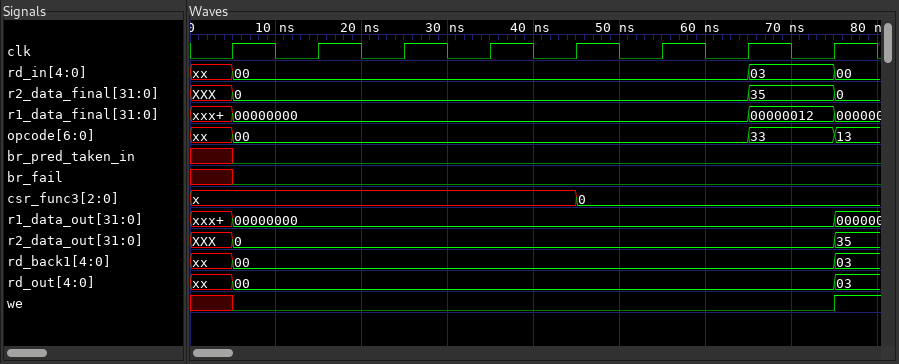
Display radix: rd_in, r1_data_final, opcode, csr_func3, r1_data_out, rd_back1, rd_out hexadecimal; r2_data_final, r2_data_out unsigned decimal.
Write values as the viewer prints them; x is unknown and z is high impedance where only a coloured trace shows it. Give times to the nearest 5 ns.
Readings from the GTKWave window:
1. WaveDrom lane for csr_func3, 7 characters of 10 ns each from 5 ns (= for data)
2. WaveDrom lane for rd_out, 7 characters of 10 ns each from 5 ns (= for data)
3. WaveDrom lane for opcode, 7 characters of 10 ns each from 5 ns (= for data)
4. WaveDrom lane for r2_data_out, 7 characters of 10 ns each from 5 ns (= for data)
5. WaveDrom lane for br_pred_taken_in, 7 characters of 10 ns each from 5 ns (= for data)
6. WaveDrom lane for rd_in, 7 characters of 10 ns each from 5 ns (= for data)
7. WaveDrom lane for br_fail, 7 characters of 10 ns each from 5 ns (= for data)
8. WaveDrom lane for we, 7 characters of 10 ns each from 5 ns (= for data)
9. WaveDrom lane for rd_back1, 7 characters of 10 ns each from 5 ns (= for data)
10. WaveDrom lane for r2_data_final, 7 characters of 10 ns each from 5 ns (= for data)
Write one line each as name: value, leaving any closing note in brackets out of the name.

WaveDrom lane for csr_func3, 7 characters of 10 ns each from 5 ns: {name: 'csr_func3', wave: 'x...=..', data: '0'}
WaveDrom lane for rd_out, 7 characters of 10 ns each from 5 ns: {name: 'rd_out', wave: '=......', data: '00'}
WaveDrom lane for opcode, 7 characters of 10 ns each from 5 ns: {name: 'opcode', wave: '=.....=', data: '00 33'}
WaveDrom lane for r2_data_out, 7 characters of 10 ns each from 5 ns: {name: 'r2_data_out', wave: '=......', data: '0'}
WaveDrom lane for br_pred_taken_in, 7 characters of 10 ns each from 5 ns: {name: 'br_pred_taken_in', wave: '0......'}
WaveDrom lane for rd_in, 7 characters of 10 ns each from 5 ns: {name: 'rd_in', wave: '=.....=', data: '00 03'}
WaveDrom lane for br_fail, 7 characters of 10 ns each from 5 ns: {name: 'br_fail', wave: '0......'}
WaveDrom lane for we, 7 characters of 10 ns each from 5 ns: {name: 'we', wave: '0......'}
WaveDrom lane for rd_back1, 7 characters of 10 ns each from 5 ns: {name: 'rd_back1', wave: '=......', data: '00'}
WaveDrom lane for r2_data_final, 7 characters of 10 ns each from 5 ns: {name: 'r2_data_final', wave: '=.....=', data: '0 35'}
